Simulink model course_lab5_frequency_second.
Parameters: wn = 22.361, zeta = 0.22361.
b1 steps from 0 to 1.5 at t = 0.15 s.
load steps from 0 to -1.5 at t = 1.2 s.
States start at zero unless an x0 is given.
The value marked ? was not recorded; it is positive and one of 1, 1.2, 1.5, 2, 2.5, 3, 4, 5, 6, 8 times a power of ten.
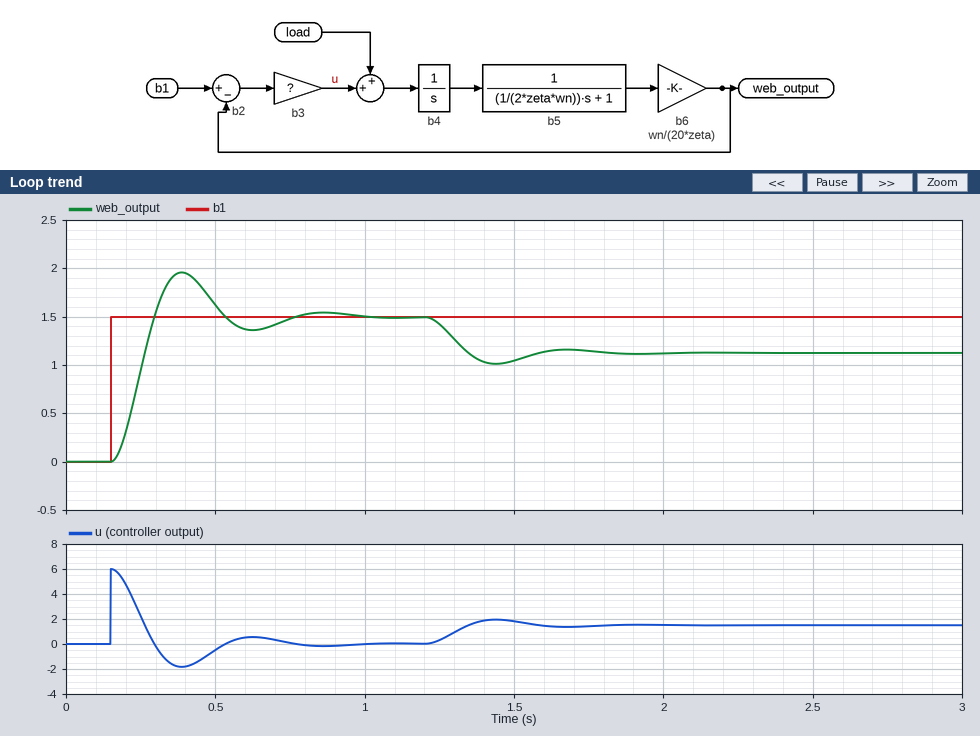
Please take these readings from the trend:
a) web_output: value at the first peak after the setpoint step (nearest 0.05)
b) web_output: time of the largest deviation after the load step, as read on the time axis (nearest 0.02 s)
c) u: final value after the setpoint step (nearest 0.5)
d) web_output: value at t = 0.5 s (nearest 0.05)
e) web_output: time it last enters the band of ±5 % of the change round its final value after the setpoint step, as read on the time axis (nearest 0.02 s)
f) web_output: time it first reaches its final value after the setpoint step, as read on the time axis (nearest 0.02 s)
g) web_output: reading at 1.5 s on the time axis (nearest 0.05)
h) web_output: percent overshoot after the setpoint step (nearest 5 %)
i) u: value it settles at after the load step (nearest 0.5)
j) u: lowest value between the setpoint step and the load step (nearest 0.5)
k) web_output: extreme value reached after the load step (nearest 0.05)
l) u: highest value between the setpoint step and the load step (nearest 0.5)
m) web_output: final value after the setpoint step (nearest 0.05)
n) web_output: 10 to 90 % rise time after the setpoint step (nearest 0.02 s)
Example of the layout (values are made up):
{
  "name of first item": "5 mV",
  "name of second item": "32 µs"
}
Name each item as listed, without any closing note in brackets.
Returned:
{
  "web_output: value at the first peak after the setpoint step": "1.95",
  "web_output: time of the largest deviation after the load step, as read on the time axis": "1.44 s",
  "u: final value after the setpoint step": "0.0",
  "web_output: value at t = 0.5 s": "1.60",
  "web_output: time it last enters the band of ±5 % of the change round its final value after the setpoint step, as read on the time axis": "0.70 s",
  "web_output: time it first reaches its final value after the setpoint step, as read on the time axis": "0.30 s",
  "web_output: reading at 1.5 s on the time axis": "1.05",
  "web_output: percent overshoot after the setpoint step": "30 %",
  "u: value it settles at after the load step": "1.5",
  "u: lowest value between the setpoint step and the load step": "-2.0",
  "web_output: extreme value reached after the load step": "1.00",
  "u: highest value between the setpoint step and the load step": "6.0",
  "web_output: final value after the setpoint step": "1.50",
  "web_output: 10 to 90 % rise time after the setpoint step": "0.10 s"
}
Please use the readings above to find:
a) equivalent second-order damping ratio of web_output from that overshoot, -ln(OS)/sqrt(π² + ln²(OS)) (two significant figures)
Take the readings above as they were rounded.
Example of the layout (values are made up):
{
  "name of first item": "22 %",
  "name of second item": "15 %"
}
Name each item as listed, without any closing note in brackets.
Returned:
{
  "equivalent second-order damping ratio of web_output from that overshoot, -ln(OS)/sqrt(π² + ln²(OS))": "0.36"
}
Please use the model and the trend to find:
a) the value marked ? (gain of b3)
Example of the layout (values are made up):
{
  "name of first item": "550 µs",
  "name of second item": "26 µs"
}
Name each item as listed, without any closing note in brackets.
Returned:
{
  "the value marked ?": "4"
}
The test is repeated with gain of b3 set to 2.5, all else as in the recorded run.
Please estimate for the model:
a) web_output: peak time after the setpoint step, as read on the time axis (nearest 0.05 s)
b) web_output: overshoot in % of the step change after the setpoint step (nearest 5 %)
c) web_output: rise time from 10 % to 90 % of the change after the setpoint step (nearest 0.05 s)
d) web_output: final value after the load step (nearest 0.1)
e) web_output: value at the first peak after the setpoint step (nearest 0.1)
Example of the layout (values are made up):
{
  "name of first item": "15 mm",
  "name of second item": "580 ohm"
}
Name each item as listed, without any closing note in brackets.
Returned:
{
  "web_output: peak time after the setpoint step, as read on the time axis": "0.45 s",
  "web_output: overshoot in % of the step change after the setpoint step": "20 %",
  "web_output: rise time from 10 % to 90 % of the change after the setpoint step": "0.15 s",
  "web_output: final value after the load step": "0.9",
  "web_output: value at the first peak after the setpoint step": "1.8"
}
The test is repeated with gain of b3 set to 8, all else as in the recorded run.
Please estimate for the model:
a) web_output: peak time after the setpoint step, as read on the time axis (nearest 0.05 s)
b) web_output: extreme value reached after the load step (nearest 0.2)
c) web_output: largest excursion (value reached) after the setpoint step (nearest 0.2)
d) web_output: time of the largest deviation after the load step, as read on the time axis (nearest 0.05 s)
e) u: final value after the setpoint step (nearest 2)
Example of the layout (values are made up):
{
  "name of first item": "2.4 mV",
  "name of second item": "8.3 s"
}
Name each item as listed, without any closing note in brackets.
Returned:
{
  "web_output: peak time after the setpoint step, as read on the time axis": "0.30 s",
  "web_output: extreme value reached after the load step": "1.2",
  "web_output: largest excursion (value reached) after the setpoint step": "2.2",
  "web_output: time of the largest deviation after the load step, as read on the time axis": "1.35 s",
  "u: final value after the setpoint step": "0"
}
